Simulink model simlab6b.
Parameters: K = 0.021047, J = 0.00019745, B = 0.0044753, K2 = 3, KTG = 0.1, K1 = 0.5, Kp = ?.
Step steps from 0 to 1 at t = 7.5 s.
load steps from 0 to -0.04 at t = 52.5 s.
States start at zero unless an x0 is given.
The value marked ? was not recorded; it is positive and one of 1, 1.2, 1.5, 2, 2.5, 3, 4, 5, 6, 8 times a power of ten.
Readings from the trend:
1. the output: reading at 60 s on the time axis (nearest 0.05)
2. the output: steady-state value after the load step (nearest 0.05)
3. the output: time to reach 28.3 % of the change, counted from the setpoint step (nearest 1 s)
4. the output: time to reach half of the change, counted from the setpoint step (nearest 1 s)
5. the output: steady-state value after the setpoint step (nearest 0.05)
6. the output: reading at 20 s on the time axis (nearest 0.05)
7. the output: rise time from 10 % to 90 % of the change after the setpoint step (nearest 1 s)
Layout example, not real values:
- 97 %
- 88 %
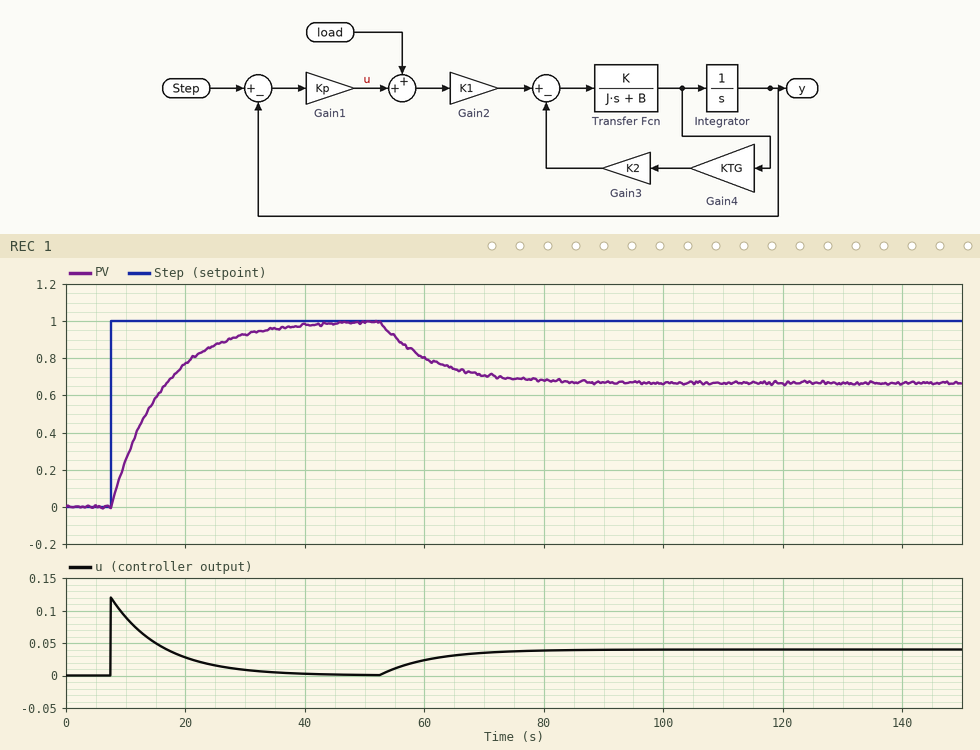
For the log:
- 0.80
- 0.65
- 3 s
- 6 s
- 1.00
- 0.75
- 19 s
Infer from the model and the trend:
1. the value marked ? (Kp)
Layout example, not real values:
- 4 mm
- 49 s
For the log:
- 0.12
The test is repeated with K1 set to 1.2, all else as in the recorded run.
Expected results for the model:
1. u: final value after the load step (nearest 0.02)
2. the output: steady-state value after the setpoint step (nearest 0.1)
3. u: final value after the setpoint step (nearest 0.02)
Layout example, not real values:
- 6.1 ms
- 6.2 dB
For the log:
- 0.04
- 1.0
- 0.00
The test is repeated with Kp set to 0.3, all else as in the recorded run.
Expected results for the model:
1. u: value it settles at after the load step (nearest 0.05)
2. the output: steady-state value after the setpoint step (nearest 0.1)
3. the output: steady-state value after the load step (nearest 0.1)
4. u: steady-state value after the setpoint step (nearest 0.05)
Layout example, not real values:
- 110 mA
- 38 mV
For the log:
- 0.05
- 1.0
- 0.9
- 0.00
